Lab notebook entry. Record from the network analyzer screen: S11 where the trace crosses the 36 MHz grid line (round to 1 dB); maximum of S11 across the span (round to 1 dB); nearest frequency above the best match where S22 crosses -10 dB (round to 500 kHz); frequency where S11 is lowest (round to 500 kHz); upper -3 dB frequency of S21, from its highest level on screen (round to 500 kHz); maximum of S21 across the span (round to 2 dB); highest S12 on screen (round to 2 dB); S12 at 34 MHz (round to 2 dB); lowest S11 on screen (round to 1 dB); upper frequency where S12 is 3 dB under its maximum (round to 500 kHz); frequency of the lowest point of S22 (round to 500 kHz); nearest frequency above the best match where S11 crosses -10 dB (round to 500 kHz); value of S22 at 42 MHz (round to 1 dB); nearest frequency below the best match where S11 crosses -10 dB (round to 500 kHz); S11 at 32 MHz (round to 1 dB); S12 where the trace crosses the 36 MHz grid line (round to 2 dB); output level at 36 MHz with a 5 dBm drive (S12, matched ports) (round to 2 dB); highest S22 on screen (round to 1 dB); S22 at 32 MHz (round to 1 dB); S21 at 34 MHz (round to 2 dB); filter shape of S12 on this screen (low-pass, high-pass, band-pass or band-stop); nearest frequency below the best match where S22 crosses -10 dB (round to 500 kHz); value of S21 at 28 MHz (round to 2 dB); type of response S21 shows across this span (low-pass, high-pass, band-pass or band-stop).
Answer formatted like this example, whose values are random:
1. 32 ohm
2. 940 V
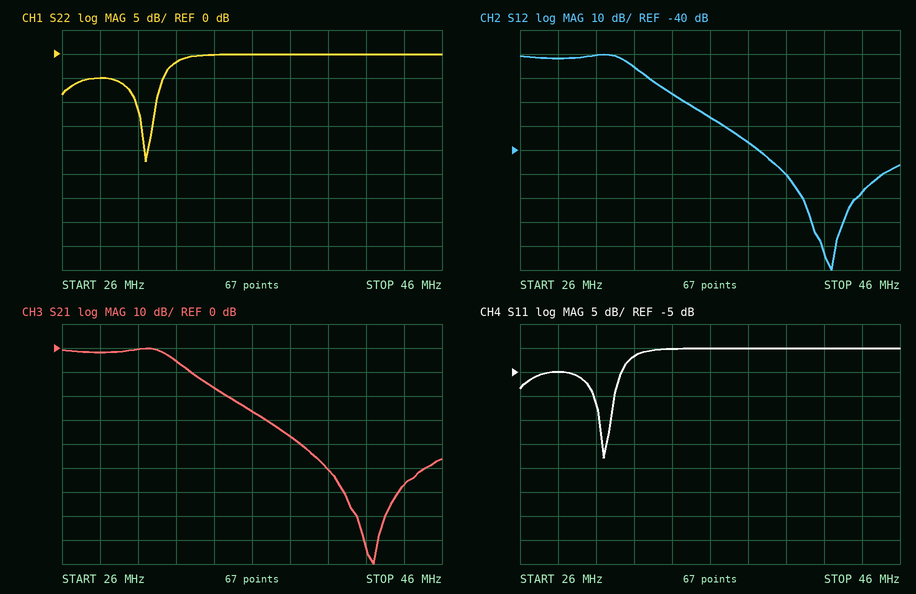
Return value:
1. 0 dB
2. 0 dB
3. 31.0 MHz
4. 30.5 MHz
5. 31.5 MHz
6. 0 dB
7. 0 dB
8. -16 dB
9. -23 dB
10. 31.5 MHz
11. 30.5 MHz
12. 31.0 MHz
13. 0 dB
14. 30.0 MHz
15. -2 dB
16. -26 dB
17. -22 dBm
18. 0 dB
19. -2 dB
20. -16 dB
21. low-pass
22. 30.0 MHz
23. -2 dB
24. low-pass
